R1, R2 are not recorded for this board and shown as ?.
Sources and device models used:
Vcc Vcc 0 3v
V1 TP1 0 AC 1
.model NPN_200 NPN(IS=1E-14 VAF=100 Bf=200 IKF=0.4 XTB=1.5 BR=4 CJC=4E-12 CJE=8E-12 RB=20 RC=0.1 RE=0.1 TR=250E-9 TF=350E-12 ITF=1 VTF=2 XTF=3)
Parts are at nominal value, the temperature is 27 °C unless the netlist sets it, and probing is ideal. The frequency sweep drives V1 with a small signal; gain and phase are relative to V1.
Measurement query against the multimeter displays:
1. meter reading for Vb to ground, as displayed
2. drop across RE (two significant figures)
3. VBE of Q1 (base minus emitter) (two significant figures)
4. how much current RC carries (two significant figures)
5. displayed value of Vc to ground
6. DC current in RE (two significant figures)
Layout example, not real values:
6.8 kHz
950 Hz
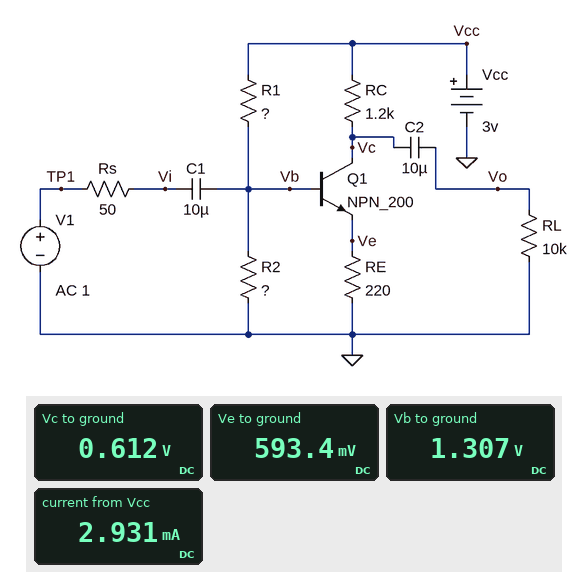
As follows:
1.307 V
590 mV
710 mV
2.0 mA
0.612 V
2.7 mA
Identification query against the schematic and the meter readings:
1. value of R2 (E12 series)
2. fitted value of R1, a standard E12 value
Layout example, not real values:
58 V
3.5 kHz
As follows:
5.6 kΩ
1.8 kΩ
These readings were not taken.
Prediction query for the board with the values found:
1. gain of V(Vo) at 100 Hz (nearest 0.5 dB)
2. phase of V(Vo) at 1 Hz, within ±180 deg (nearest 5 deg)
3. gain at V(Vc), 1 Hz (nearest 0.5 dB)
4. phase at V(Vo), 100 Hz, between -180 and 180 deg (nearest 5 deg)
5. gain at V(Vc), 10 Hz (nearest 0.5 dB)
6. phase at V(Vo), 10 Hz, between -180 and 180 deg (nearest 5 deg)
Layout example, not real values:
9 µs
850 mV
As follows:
-6.0 dB
145 deg
-40.5 dB
35 deg
-21.0 dB
90 deg
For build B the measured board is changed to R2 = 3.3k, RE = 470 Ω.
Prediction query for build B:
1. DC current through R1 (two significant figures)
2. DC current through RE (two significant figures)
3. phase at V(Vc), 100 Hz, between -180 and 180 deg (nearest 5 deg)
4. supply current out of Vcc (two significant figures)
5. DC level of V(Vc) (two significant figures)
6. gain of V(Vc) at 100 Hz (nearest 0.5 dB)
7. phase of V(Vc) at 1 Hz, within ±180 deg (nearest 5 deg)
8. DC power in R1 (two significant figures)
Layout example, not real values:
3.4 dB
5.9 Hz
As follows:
770 µA
2.0 mA
25 deg
2.5 mA
960 mV
-5.0 dB
90 deg
1.1 mW
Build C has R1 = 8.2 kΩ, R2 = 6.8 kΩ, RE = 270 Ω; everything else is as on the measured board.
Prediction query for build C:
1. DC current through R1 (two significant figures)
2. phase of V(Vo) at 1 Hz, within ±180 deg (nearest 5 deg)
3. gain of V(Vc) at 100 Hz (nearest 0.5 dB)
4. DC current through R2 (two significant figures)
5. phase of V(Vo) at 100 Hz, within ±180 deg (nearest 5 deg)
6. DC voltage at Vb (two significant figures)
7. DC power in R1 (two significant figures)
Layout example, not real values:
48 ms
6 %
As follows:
220 µA
-35 deg
-1.5 dB
180 µA
-160 deg
1.2 V
390 µW
